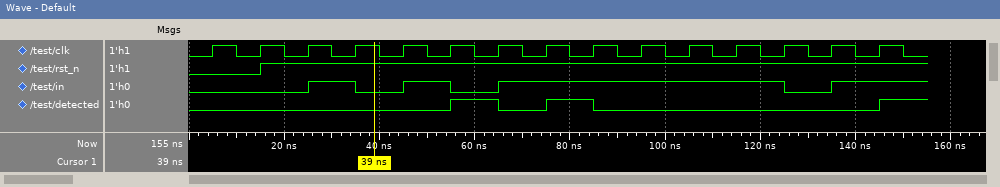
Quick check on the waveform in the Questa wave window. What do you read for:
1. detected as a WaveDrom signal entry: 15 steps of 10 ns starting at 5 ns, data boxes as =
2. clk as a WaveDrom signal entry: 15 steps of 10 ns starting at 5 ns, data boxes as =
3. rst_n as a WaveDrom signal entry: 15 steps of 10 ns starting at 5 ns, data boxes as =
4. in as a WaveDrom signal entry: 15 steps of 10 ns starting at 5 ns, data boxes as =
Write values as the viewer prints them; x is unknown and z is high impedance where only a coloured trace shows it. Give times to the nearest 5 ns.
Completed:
{name: 'detected', wave: '0....1010.....1'}
{name: 'clk', wave: 'p..............'}
{name: 'rst_n', wave: '01.............'}
{name: 'in', wave: '0.10101.....01.'}
